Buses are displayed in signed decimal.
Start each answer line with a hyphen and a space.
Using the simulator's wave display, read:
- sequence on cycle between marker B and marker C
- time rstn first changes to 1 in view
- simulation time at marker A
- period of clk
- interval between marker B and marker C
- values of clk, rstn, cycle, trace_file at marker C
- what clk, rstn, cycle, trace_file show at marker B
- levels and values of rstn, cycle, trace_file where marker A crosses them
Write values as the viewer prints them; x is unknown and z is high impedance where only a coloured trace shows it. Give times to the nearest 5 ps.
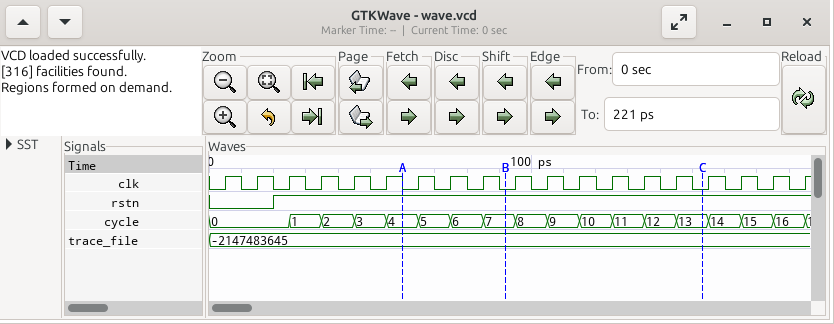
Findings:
- 7, 8, 9, 10, 11, 12, 13
- 20 ps
- 60 ps
- 10 ps
- 60 ps
- clk=0, rstn=1, cycle=13, trace_file=-2147483645
- clk=0, rstn=1, cycle=7, trace_file=-2147483645
- rstn=1, cycle=4, trace_file=-2147483645
